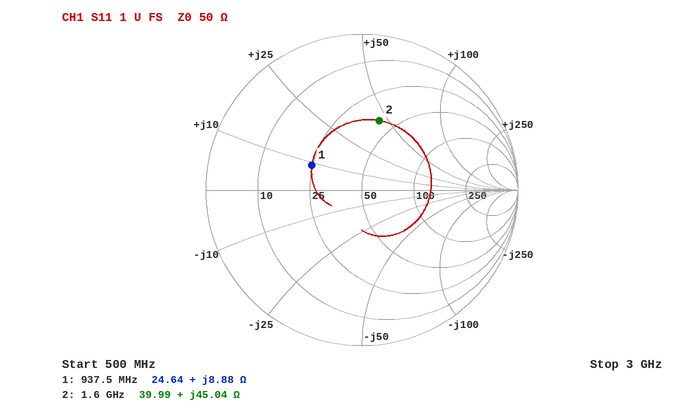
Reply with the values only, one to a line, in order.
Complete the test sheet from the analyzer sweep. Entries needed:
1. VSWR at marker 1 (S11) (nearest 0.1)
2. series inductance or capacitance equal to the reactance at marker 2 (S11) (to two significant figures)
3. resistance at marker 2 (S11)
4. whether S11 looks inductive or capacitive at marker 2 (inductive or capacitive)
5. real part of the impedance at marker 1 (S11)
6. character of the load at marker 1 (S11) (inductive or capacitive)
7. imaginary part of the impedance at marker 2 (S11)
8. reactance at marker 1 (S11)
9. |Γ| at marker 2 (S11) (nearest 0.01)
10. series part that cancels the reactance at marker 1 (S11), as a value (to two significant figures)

2.1
4.5 nH
39.99 Ω
inductive
24.64 Ω
inductive
+45.04 Ω
+8.88 Ω
0.46
19 pF
